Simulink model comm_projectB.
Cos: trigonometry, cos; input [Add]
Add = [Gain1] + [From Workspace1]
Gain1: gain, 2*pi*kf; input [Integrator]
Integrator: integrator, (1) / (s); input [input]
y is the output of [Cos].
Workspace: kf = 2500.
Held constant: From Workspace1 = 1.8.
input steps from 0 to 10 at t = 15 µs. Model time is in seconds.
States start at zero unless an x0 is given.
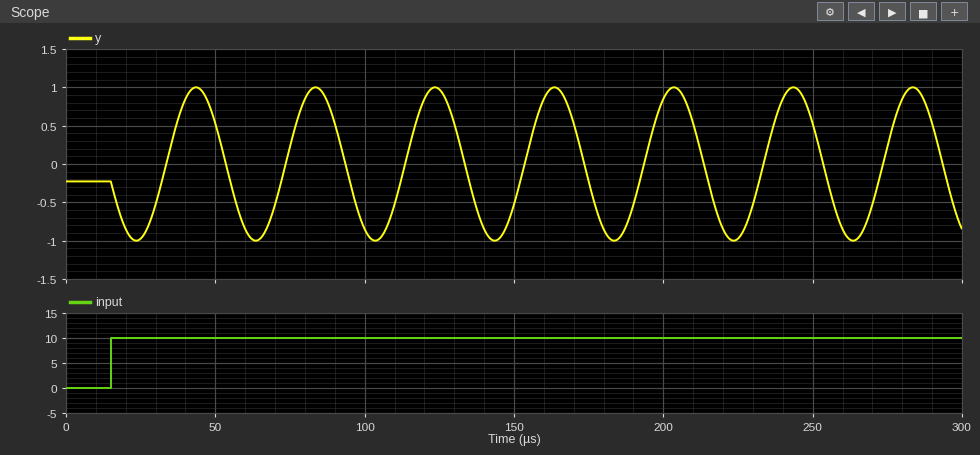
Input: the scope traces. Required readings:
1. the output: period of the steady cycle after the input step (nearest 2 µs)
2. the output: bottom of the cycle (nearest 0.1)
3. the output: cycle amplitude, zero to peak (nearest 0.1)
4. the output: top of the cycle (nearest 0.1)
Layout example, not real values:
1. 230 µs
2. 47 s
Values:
1. 40 µs
2. -1.0
3. 1.0
4. 1.0
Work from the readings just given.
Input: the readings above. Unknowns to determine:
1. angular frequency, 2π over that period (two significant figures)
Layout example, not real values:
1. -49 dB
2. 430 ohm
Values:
1. 0.16 rad/µs
